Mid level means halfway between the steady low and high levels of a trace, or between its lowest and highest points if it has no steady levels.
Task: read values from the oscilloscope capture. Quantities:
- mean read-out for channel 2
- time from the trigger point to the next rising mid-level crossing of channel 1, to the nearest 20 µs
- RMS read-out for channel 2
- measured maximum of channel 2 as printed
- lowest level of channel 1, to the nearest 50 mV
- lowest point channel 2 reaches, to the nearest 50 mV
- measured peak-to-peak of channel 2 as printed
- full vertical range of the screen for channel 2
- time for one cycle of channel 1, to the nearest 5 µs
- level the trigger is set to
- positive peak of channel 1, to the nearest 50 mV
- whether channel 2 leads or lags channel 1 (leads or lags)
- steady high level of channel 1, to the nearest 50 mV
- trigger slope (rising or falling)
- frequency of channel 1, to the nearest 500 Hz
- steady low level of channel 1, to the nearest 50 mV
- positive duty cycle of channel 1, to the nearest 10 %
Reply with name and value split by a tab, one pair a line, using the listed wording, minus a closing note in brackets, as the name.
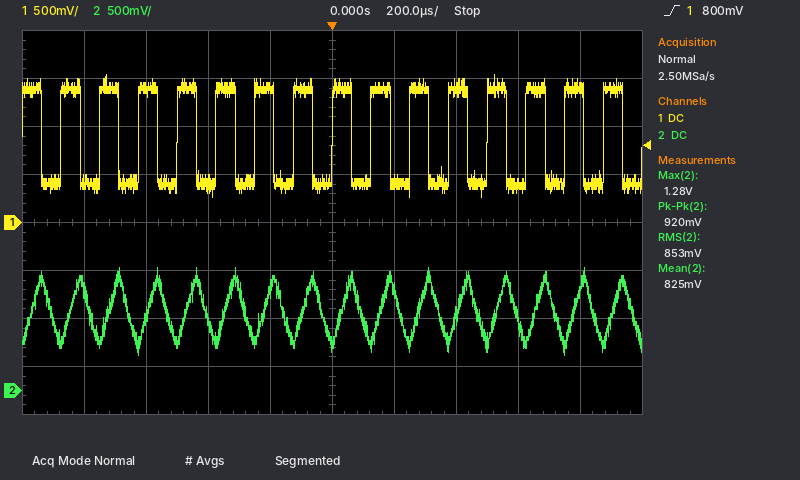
mean read-out for channel 2	825 mV
time from the trigger point to the next rising mid-level crossing of channel 1, to the nearest 20 µs	120 µs
RMS read-out for channel 2	853 mV
measured maximum of channel 2 as printed	1.28 V
lowest level of channel 1, to the nearest 50 mV	250 mV
lowest point channel 2 reaches, to the nearest 50 mV	350 mV
measured peak-to-peak of channel 2 as printed	920 mV
full vertical range of the screen for channel 2	4 V
time for one cycle of channel 1, to the nearest 5 µs	125 µs
level the trigger is set to	800 mV
positive peak of channel 1, to the nearest 50 mV	1.55 V
whether channel 2 leads or lags channel 1	lags
steady high level of channel 1, to the nearest 50 mV	1.40 V
trigger slope	rising
frequency of channel 1, to the nearest 500 Hz	8.0 kHz
steady low level of channel 1, to the nearest 50 mV	400 mV
positive duty cycle of channel 1, to the nearest 10 %	50 %
